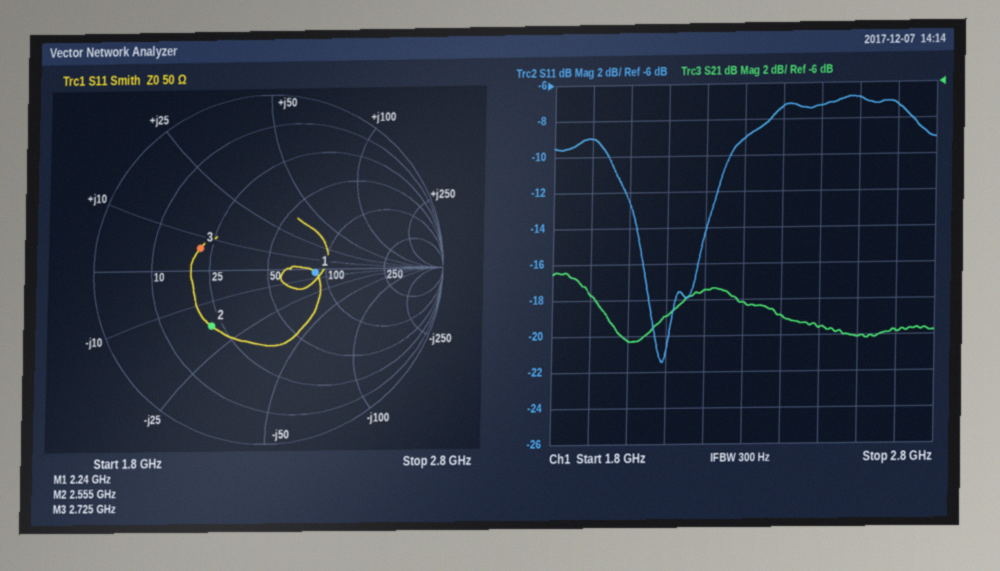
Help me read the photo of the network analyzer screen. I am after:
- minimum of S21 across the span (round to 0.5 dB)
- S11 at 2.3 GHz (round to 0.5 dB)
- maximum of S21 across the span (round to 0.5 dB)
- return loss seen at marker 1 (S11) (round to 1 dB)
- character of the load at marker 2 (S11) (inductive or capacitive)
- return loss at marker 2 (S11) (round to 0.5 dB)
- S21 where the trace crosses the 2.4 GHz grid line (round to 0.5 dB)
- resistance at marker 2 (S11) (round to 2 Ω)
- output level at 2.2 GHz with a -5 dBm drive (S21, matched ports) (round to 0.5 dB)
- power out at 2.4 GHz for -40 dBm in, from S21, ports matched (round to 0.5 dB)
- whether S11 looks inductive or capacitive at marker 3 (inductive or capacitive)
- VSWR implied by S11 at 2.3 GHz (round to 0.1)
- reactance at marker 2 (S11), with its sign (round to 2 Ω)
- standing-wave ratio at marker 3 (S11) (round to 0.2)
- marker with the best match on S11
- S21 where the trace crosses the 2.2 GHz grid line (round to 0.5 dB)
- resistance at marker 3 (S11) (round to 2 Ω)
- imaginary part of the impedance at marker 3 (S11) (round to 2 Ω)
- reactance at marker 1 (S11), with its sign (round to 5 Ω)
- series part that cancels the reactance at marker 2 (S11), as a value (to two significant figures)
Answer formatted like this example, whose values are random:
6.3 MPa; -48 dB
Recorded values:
-20.5 dB; -9.0 dB; -16.5 dB; 11 dB; capacitive; 7.0 dB; -19.0 dB; 22 Ω; -22.5 dBm; -59.0 dBm; inductive; 2.1; -18 Ω; 2.4; marker 1; -17.5 dB; 22 Ω; +6 Ω; -5 Ω; 1.1 nH
